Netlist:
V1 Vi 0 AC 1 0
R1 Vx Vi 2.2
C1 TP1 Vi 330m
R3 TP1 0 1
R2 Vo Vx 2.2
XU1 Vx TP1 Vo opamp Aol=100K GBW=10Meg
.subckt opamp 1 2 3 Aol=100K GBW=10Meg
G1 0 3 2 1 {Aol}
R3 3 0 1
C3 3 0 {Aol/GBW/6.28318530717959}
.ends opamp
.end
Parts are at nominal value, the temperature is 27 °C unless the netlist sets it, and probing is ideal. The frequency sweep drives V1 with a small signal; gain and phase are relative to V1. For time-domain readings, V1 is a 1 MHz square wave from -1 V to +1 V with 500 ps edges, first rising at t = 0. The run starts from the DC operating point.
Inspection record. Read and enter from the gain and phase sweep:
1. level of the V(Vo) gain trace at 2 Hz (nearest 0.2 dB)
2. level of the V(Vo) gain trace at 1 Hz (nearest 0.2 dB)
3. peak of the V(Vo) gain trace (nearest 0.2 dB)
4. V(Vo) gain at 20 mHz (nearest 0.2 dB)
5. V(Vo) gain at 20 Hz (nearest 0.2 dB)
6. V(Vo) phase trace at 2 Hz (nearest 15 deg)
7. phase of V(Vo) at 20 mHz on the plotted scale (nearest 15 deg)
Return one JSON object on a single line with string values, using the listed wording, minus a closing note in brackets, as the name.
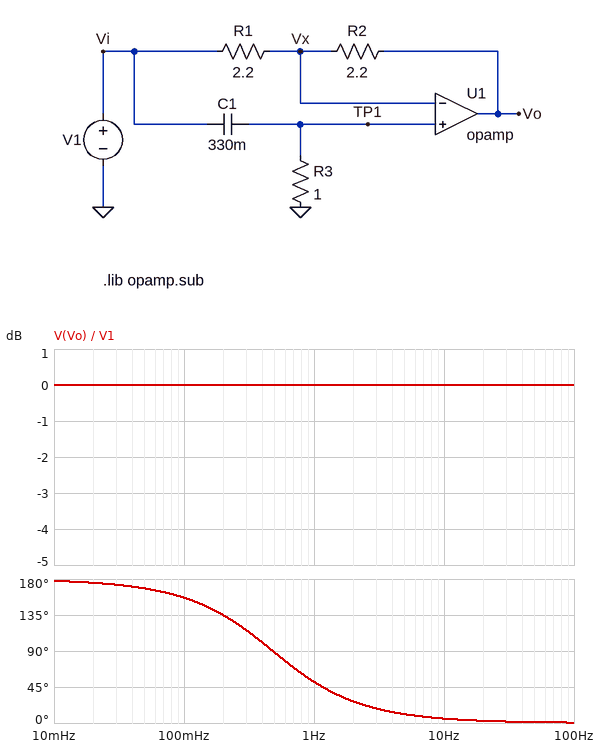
{"level of the V(Vo) gain trace at 2 Hz": "0 dB", "level of the V(Vo) gain trace at 1 Hz": "0 dB", "peak of the V(Vo) gain trace": "0 dB", "V(Vo) gain at 20 mHz": "0 dB", "V(Vo) gain at 20 Hz": "0 dB", "V(Vo) phase trace at 2 Hz": "30 deg", "phase of V(Vo) at 20 mHz on the plotted scale": "180 deg"}
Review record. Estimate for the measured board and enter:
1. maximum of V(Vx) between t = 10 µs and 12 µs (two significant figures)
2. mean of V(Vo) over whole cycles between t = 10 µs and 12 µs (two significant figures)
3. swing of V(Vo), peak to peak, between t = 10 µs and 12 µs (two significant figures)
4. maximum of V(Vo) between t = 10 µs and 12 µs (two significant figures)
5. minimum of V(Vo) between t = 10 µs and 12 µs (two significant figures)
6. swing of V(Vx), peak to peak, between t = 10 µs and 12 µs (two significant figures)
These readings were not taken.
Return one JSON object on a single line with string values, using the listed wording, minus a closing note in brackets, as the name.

{"maximum of V(Vx) between t = 10 µs and 12 µs": "2.0 V", "mean of V(Vo) over whole cycles between t = 10 µs and 12 µs": "2.0 V", "swing of V(Vo), peak to peak, between t = 10 µs and 12 µs": "2.0 V", "maximum of V(Vo) between t = 10 µs and 12 µs": "3.0 V", "minimum of V(Vo) between t = 10 µs and 12 µs": "1.0 V", "swing of V(Vx), peak to peak, between t = 10 µs and 12 µs": "2.0 V"}
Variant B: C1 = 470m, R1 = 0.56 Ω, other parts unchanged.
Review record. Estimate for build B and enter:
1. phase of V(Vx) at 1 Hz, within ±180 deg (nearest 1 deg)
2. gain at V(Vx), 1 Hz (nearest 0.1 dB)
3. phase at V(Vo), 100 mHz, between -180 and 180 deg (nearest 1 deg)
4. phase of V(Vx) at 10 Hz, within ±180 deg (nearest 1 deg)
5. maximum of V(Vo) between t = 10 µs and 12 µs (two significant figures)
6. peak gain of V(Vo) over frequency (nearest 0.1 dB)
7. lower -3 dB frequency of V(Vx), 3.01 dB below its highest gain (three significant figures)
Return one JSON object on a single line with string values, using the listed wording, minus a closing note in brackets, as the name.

{"phase of V(Vx) at 1 Hz, within ±180 deg": "19 deg", "gain at V(Vx), 1 Hz": "-0.5 dB", "phase at V(Vo), 100 mHz, between -180 and 180 deg": "159 deg", "phase of V(Vx) at 10 Hz, within ±180 deg": "2 deg", "maximum of V(Vo) between t = 10 µs and 12 µs": "5.9 V", "peak gain of V(Vo) over frequency": "11.9 dB", "lower -3 dB frequency of V(Vx), 3.01 dB below its highest gain": "339 mHz"}
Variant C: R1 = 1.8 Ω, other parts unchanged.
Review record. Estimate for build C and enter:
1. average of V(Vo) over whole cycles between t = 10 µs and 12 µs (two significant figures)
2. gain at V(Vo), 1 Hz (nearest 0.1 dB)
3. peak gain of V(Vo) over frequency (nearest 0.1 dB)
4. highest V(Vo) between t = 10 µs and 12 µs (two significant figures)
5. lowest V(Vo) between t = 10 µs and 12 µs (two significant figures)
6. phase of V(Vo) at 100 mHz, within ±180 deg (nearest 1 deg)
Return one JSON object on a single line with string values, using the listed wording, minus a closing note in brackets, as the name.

{"average of V(Vo) over whole cycles between t = 10 µs and 12 µs": "2.2 V", "gain at V(Vo), 1 Hz": "0.4 dB", "peak gain of V(Vo) over frequency": "1.7 dB", "highest V(Vo) between t = 10 µs and 12 µs": "3.2 V", "lowest V(Vo) between t = 10 µs and 12 µs": "1.2 V", "phase of V(Vo) at 100 mHz, within ±180 deg": "159 deg"}
